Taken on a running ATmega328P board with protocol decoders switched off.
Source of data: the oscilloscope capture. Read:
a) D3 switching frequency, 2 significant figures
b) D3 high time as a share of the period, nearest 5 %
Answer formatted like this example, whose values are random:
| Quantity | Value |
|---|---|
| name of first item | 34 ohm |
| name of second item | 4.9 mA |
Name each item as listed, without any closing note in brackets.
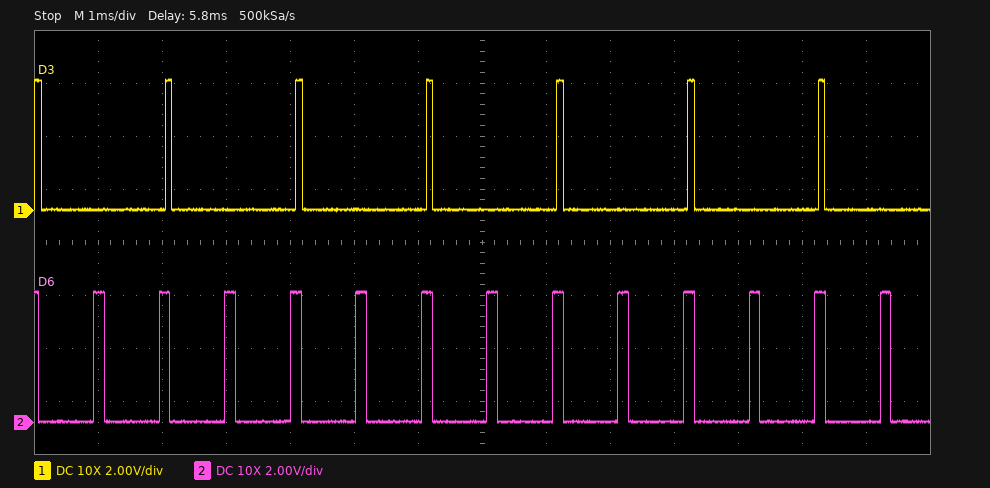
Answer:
| Quantity | Value |
|---|---|
| D3 switching frequency, 2 significant figures | 490 Hz |
| D3 high time as a share of the period, nearest 5 % | 5 % |
